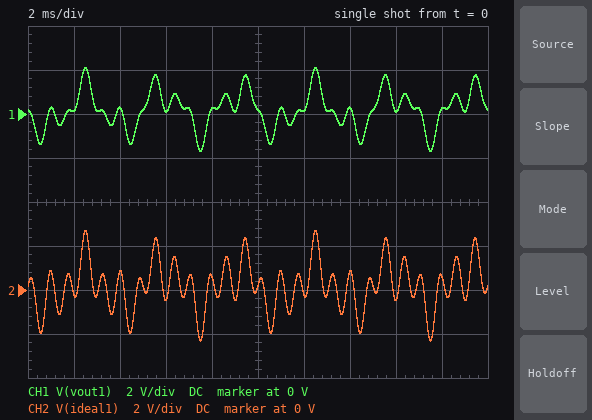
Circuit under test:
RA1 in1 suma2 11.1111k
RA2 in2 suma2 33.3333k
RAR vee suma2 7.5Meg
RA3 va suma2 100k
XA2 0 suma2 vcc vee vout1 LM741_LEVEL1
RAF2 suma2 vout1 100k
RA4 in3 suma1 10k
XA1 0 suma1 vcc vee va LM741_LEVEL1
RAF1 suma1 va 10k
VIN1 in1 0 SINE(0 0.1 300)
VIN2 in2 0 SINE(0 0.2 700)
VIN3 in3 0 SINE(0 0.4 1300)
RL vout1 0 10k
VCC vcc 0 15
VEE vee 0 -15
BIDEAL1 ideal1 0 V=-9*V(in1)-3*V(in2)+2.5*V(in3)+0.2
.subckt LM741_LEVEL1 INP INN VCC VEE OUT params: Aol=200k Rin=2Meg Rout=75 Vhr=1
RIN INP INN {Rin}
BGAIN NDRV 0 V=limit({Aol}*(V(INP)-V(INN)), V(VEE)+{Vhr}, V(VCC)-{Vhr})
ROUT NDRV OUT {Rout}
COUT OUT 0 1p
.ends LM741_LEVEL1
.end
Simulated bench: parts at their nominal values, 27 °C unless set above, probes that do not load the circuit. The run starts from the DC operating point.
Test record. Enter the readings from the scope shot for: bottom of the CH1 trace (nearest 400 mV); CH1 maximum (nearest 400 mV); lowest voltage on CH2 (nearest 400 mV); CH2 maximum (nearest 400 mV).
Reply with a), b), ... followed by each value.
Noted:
a) -1.6 V
b) 2.0 V
c) -2.4 V
d) 2.8 V
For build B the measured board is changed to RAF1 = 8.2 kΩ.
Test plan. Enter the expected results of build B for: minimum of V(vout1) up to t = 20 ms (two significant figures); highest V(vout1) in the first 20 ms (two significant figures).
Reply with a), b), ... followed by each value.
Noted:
a) -1.6 V
b) 2.0 V
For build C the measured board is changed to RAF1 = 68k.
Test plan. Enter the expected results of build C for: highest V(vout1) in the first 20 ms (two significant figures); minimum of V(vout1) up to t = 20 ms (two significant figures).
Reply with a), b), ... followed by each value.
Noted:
a) 4.4 V
b) -4.0 V
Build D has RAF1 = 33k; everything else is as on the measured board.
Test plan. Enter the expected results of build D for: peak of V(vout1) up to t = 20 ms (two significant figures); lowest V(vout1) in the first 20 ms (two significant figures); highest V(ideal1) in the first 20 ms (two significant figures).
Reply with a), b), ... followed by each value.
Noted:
a) 3.0 V
b) -2.6 V
c) 2.7 V
